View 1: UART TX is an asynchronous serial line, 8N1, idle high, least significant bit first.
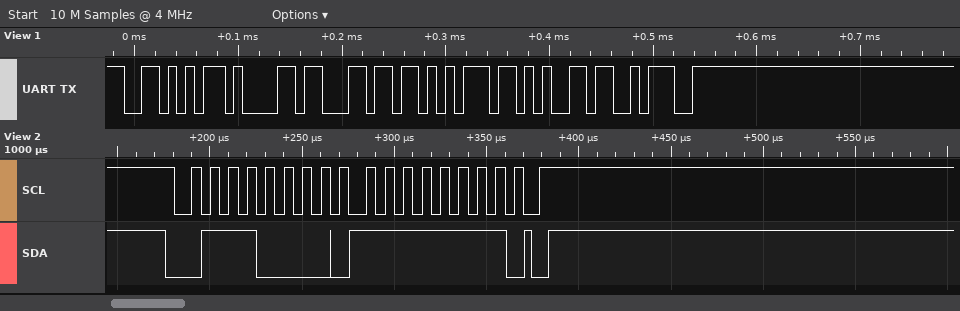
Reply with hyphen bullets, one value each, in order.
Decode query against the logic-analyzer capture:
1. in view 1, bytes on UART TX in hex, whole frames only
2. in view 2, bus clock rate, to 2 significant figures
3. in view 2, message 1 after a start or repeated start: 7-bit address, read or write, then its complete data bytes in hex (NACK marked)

- 56 61 6C 75 65 3A
- 100 kHz
- 0x38 write: FF
